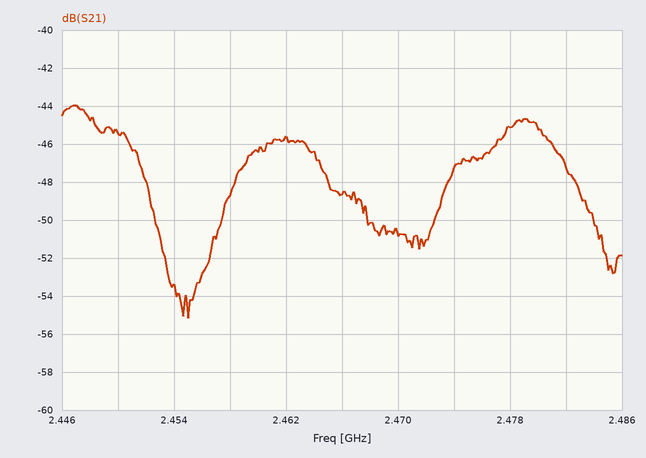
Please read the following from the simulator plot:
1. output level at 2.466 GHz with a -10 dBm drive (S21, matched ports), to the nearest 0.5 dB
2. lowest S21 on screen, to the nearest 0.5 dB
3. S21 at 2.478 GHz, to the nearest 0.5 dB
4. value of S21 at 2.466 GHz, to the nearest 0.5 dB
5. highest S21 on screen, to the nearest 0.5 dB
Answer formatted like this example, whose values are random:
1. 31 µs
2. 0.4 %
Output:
1. -58.5 dBm
2. -55.0 dB
3. -45.0 dB
4. -48.5 dB
5. -44.0 dB
